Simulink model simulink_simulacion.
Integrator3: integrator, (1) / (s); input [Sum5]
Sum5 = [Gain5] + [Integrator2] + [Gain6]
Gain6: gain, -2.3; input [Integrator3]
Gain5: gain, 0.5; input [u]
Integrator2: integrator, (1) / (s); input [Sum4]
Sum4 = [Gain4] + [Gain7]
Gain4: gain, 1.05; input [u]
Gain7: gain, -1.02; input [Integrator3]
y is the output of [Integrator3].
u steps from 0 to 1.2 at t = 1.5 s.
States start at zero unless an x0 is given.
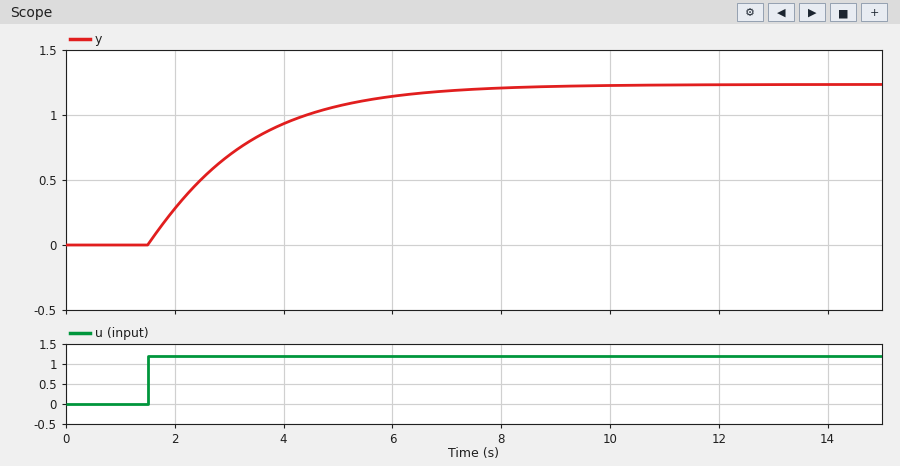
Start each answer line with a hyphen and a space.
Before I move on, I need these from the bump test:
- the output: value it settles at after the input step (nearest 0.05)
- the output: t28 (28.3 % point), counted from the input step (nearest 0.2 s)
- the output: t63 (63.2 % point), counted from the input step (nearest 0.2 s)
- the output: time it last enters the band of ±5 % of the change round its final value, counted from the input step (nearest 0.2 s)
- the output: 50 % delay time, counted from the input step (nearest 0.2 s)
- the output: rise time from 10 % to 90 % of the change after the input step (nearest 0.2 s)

- 1.25
- 0.6 s
- 1.8 s
- 5.2 s
- 1.2 s
- 3.8 s
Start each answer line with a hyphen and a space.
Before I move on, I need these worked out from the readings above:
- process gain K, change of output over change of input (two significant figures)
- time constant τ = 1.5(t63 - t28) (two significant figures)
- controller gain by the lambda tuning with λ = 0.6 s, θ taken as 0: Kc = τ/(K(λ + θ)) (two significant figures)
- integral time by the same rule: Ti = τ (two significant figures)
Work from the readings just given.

- 1.0
- 1.8 s
- 3.0
- 1.8 s
